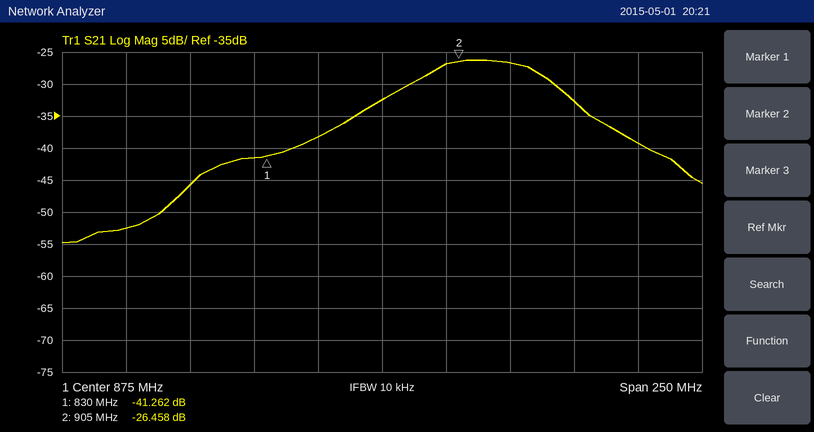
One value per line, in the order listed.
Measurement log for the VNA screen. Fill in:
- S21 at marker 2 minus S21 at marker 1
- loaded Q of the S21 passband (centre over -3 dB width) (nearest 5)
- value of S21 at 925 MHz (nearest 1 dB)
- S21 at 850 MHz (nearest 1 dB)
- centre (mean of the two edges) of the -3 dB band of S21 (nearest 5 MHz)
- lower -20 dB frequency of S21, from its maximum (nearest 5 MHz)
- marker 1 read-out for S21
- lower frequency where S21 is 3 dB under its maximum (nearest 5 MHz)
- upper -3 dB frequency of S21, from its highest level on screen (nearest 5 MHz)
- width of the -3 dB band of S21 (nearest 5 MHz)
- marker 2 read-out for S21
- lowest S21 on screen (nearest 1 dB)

14.804 dB
20
-27 dB
-38 dB
915 MHz
800 MHz
-41.262 dB
890 MHz
940 MHz
50 MHz
-26.458 dB
-55 dB
